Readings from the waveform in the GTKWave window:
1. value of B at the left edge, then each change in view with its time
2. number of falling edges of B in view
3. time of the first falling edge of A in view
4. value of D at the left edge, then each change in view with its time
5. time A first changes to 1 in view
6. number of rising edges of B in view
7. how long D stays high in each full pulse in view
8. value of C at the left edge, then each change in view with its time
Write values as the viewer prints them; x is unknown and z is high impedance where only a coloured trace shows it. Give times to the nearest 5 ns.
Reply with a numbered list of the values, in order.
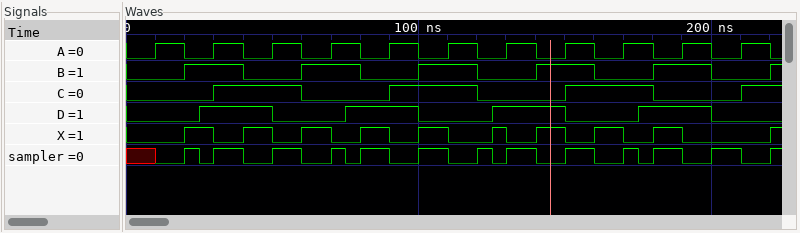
1. 0, 1 at 20 ns, 0 at 40 ns, 1 at 60 ns, 0 at 80 ns, 1 at 100 ns, 0 at 120 ns, 1 at 140 ns, 0 at 160 ns, 1 at 180 ns, 0 at 200 ns, 1 at 220 ns
2. 5
3. 20 ns
4. 0, 1 at 25 ns, 0 at 50 ns, 1 at 75 ns, 0 at 100 ns, 1 at 125 ns, 0 at 150 ns, 1 at 175 ns, 0 at 200 ns
5. 10 ns
6. 6
7. 25 ns, 25 ns, 25 ns, 25 ns
8. 0, 1 at 30 ns, 0 at 60 ns, 1 at 90 ns, 0 at 120 ns, 1 at 150 ns, 0 at 180 ns, 1 at 210 ns
